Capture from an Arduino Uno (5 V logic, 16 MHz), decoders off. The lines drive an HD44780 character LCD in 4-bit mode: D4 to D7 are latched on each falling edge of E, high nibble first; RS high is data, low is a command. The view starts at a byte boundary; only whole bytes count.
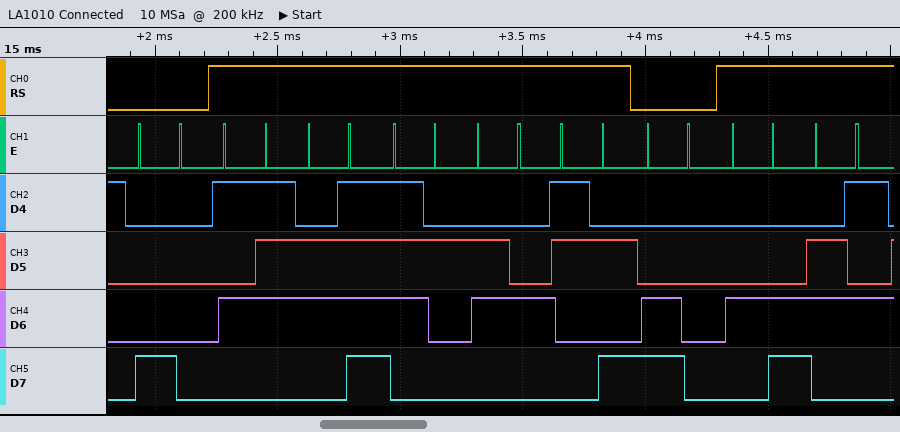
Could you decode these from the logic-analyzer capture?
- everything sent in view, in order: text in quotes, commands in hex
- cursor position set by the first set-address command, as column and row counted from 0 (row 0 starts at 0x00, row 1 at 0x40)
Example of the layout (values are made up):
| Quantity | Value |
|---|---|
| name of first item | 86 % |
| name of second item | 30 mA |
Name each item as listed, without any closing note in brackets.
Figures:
| Quantity | Value |
|---|---|
| everything sent in view, in order: text in quotes, commands in hex | 0x80 "Word:" 0xC0 "Le" |
| cursor position set by the first set-address command, as column and row counted from 0 | column 0, row 0 |
